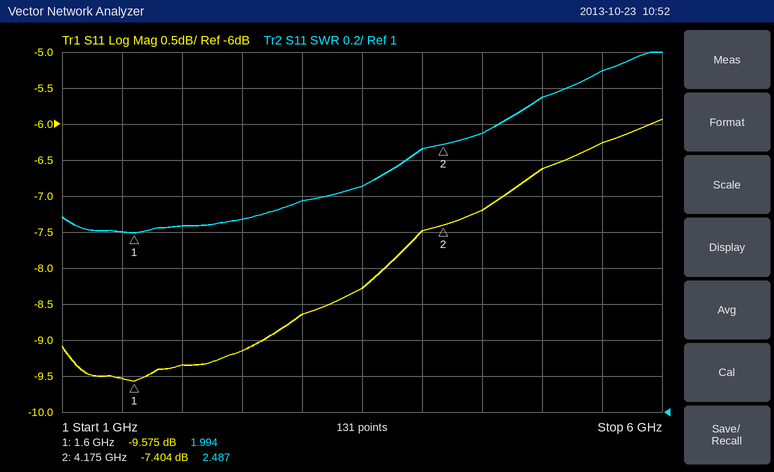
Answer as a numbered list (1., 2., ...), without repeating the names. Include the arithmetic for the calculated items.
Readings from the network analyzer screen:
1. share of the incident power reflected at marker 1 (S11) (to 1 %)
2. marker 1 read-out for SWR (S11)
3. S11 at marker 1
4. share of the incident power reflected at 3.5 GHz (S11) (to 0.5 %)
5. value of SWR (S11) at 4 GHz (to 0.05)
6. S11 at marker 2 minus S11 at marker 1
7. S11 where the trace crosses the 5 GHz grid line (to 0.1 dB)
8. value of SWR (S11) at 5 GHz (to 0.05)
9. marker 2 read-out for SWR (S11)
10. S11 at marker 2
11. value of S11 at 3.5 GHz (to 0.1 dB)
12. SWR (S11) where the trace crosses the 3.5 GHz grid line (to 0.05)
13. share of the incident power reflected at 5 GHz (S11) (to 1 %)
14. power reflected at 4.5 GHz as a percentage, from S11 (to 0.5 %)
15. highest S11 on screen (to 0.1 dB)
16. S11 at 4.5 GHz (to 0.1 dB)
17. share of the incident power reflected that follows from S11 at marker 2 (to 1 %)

1. 10^(-9.575/10) ≈ 11 %
2. 1.994
3. -9.575 dB
4. 10^(-8.3/10) ≈ 14.8 %, so 15.0 % to the nearest 0.5 %
5. 2.45
6. -7.404 − (-9.575) = 2.171 dB
7. -6.6 dB
8. 2.75
9. 2.487
10. -7.404 dB
11. -8.3 dB
12. 2.25
13. 10^(-6.6/10) ≈ 22 %
14. 10^(-7.2/10) ≈ 19.1 %, so 19.0 % to the nearest 0.5 %
15. -5.9 dB
16. -7.2 dB
17. 10^(-7.404/10) ≈ 18 %
